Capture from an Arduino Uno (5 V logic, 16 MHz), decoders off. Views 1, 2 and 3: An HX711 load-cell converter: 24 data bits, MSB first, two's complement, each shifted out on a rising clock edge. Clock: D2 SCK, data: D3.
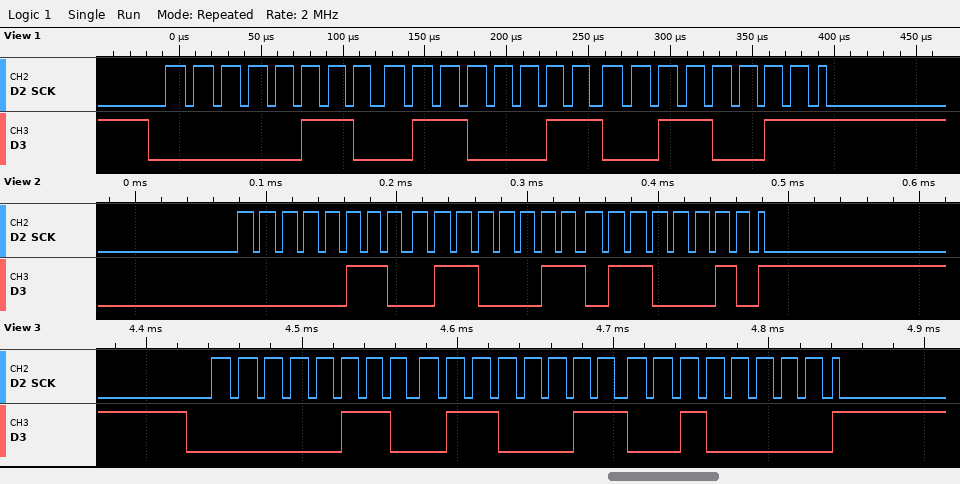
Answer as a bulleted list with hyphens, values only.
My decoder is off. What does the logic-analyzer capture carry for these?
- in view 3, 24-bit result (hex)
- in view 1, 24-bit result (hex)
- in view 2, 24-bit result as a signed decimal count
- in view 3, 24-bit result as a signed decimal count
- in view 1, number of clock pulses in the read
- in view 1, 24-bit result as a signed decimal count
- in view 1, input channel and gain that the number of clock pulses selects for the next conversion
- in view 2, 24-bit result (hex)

- 0x066320
- 0x066333
- 418658
- 418592
- 25
- 418611
- channel A, gain 128
- 0x066362
